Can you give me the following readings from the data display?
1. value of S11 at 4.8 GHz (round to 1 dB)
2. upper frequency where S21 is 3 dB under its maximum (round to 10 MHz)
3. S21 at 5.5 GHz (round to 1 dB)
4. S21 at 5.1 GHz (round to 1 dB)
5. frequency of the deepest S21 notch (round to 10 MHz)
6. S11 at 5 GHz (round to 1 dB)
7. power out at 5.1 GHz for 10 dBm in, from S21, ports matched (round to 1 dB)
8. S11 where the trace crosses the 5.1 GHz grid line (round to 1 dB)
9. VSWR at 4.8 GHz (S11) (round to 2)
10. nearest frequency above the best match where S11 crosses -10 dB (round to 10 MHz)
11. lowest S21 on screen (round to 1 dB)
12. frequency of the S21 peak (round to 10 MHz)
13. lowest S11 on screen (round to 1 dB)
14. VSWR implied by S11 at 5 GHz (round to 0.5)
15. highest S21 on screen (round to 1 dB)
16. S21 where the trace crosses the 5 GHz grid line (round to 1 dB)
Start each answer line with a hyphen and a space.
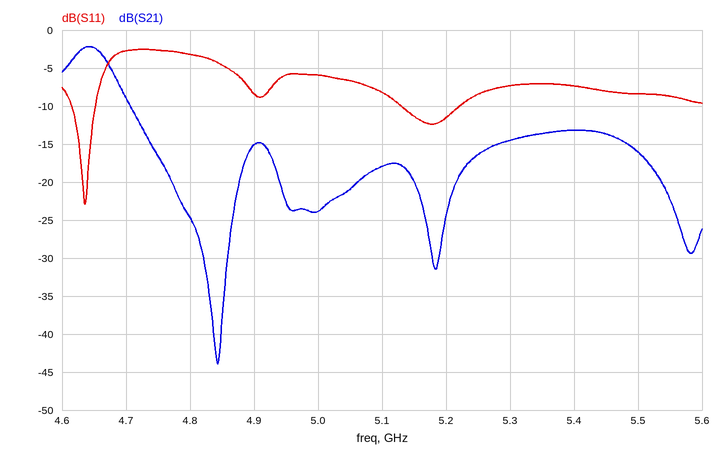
- -3 dB
- 4.68 GHz
- -16 dB
- -18 dB
- 4.84 GHz
- -6 dB
- -8 dBm
- -8 dB
- 6
- 4.65 GHz
- -44 dB
- 4.64 GHz
- -23 dB
- 3.0
- -2 dB
- -24 dB
